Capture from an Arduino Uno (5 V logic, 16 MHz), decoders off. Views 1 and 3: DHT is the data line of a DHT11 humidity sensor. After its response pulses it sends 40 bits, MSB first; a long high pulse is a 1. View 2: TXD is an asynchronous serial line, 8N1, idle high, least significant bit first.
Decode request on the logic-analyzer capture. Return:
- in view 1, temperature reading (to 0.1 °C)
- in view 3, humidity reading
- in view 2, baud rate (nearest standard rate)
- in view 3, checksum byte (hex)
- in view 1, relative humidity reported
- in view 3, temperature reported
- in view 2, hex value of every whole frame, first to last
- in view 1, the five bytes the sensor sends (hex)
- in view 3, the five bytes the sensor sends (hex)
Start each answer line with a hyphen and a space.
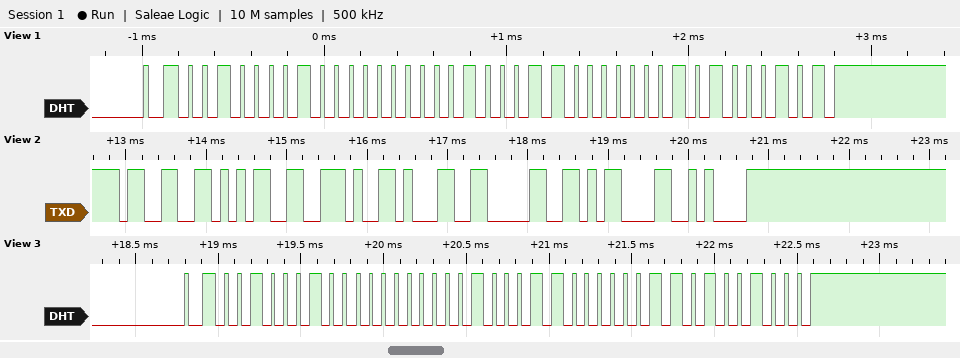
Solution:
- 35.1 °C
- 34 %
- 9600 baud
- 0x48
- 33 %
- 35.3 °C
- 0x33 0x35 0x2E 0x31 0x30 0x0D 0x0A
- 21 00 23 01 45
- 22 00 23 03 48
